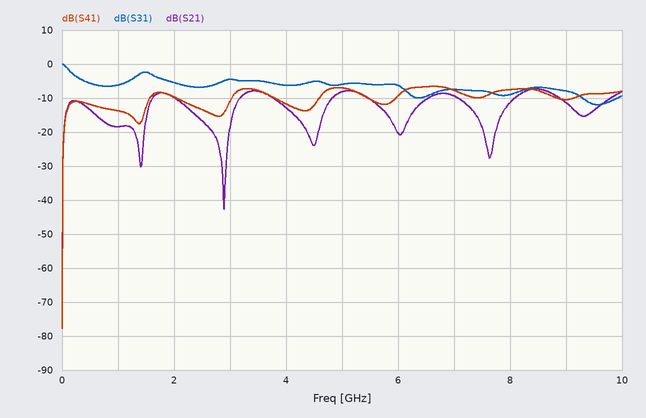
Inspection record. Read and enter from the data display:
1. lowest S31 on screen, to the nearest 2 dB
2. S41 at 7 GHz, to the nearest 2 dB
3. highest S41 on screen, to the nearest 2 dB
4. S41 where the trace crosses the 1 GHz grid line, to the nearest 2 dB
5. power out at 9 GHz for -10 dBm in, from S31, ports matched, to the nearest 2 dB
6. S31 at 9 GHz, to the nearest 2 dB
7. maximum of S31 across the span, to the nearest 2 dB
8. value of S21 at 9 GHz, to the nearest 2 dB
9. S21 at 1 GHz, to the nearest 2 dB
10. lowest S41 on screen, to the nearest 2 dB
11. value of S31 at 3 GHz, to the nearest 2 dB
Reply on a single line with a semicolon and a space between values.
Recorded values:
-12 dB; -8 dB; -6 dB; -14 dB; -18 dBm; -8 dB; 0 dB; -12 dB; -18 dB; -78 dB; -4 dB
